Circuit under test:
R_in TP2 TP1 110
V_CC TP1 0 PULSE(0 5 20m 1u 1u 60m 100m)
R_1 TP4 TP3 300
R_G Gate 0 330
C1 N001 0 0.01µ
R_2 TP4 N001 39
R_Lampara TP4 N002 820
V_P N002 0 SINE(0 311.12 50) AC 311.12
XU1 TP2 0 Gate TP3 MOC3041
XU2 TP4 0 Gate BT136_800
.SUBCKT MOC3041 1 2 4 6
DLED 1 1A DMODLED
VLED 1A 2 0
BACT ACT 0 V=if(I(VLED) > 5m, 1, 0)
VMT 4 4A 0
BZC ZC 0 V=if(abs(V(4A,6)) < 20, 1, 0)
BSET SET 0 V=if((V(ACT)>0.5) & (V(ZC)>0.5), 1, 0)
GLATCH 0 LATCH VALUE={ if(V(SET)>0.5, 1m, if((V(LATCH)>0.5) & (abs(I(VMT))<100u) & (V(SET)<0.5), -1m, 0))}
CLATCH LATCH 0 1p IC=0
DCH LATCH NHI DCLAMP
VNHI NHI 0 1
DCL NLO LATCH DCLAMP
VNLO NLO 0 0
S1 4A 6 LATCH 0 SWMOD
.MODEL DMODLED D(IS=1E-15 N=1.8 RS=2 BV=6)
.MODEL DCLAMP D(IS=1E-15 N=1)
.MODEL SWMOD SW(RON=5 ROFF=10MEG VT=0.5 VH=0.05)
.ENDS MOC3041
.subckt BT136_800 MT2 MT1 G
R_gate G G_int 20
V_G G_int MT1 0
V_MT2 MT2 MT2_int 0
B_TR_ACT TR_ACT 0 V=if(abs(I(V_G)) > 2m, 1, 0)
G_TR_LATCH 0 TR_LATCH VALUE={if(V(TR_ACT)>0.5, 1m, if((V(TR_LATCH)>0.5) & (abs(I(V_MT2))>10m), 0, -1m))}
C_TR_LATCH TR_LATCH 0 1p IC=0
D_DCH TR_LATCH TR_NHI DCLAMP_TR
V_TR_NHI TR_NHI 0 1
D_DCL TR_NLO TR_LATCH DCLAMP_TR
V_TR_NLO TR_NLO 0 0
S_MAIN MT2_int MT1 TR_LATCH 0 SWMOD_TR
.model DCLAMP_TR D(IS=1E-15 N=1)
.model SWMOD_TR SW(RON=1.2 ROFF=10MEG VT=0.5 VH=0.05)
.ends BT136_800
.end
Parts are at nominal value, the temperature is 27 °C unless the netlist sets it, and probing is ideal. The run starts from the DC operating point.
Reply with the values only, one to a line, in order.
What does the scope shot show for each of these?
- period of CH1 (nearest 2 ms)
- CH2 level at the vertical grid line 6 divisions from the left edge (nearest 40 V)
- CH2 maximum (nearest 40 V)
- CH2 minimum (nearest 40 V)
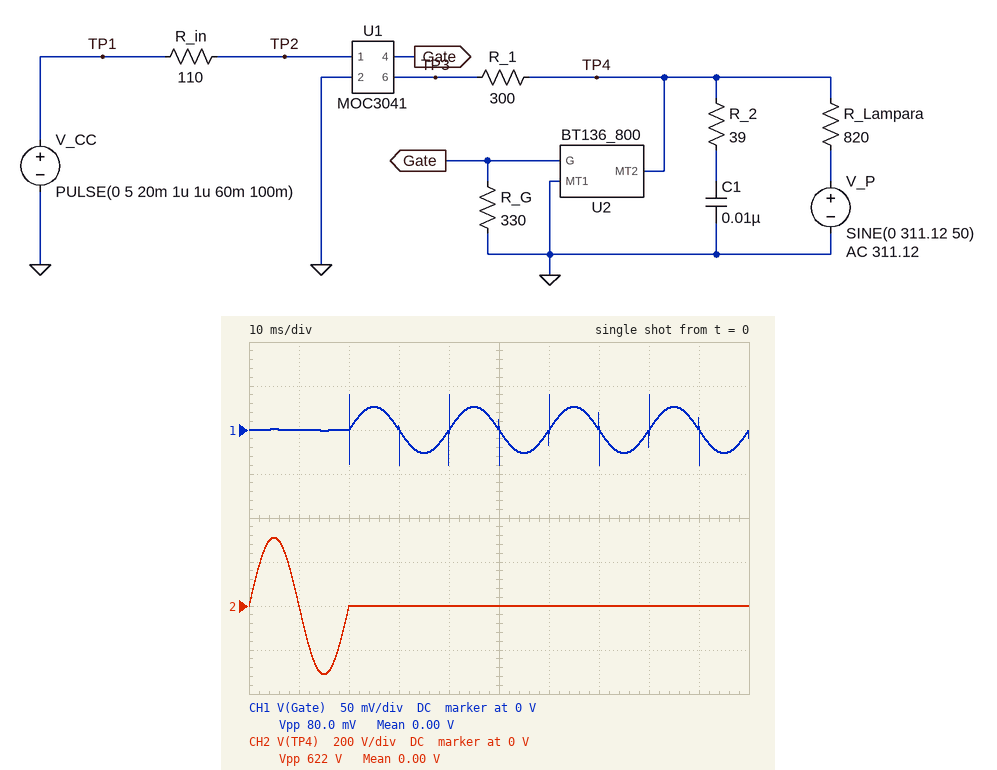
20 ms
0 V
320 V
-320 V
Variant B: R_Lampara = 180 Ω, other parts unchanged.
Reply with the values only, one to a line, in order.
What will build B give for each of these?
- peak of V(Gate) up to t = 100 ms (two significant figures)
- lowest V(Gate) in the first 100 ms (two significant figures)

120 mV
-120 mV
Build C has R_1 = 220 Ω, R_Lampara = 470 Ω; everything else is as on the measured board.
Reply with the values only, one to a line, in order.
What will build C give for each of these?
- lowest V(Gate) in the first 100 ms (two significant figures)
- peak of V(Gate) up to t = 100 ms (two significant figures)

-61 mV
61 mV
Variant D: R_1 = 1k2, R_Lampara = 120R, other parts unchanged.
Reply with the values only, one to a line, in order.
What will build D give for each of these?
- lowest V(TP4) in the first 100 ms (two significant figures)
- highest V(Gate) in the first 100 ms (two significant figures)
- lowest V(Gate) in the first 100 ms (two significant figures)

-310 V
47 mV
-47 mV
